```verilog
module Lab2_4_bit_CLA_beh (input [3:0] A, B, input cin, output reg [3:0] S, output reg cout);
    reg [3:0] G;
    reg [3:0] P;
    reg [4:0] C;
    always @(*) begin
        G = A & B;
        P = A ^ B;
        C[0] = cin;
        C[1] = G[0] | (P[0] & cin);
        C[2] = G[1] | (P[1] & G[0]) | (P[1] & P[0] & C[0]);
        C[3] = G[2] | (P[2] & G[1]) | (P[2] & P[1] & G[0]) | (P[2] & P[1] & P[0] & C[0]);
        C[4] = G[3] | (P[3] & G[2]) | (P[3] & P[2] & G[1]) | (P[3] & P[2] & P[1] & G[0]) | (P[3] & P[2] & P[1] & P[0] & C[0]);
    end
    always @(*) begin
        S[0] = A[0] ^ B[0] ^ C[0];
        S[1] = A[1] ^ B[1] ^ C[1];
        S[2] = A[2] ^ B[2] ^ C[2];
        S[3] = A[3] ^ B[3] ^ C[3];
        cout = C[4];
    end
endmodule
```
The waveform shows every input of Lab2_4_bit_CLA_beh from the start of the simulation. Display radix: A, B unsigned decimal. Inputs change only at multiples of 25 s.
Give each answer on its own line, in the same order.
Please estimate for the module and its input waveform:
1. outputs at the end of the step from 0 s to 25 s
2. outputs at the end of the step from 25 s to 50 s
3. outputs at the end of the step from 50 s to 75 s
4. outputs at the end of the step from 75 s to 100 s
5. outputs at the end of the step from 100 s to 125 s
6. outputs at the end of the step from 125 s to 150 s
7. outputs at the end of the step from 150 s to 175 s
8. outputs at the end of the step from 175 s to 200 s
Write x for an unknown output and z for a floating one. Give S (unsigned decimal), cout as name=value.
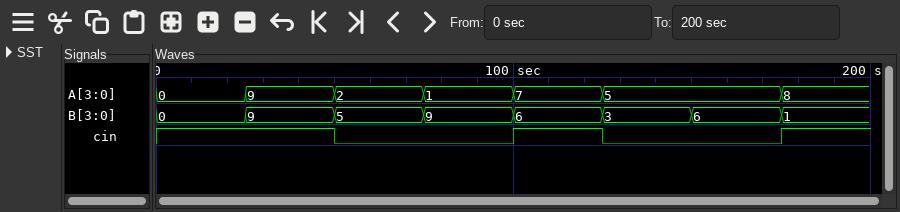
S=1, cout=0
S=3, cout=1
S=7, cout=0
S=10, cout=0
S=14, cout=0
S=8, cout=0
S=11, cout=0
S=10, cout=0
